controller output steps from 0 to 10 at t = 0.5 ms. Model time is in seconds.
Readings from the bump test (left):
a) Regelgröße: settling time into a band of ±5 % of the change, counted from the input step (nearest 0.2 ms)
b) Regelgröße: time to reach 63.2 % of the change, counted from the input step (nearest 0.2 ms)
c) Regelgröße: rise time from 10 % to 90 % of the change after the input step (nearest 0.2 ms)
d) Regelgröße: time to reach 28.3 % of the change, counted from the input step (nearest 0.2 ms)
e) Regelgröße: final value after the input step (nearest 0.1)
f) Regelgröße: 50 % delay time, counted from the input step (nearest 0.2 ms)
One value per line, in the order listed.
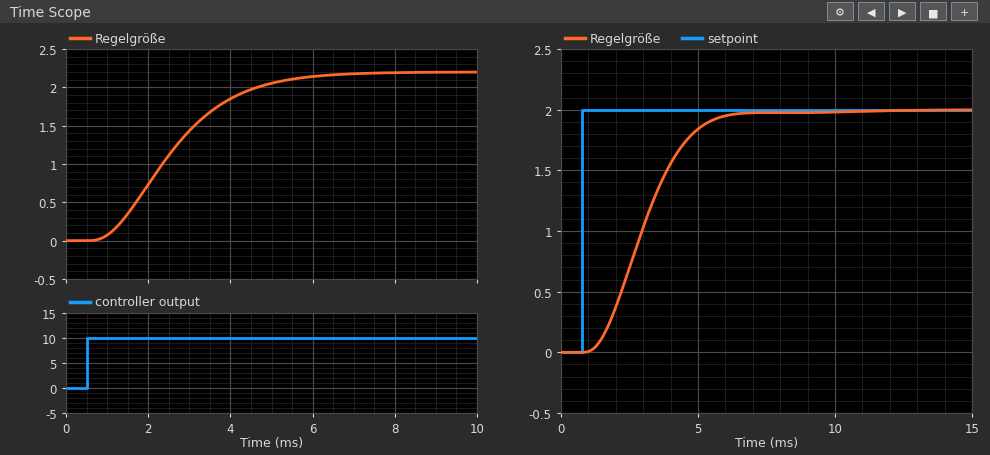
4.8 ms
2.4 ms
3.2 ms
1.4 ms
2.2
2.0 ms
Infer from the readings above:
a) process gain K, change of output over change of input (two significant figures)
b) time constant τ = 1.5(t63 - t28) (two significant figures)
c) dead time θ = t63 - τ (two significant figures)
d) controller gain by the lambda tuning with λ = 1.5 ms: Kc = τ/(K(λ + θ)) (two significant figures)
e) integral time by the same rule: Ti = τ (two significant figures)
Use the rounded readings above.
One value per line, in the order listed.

0.22
1.5 ms
0.90 ms
2.8
1.5 ms
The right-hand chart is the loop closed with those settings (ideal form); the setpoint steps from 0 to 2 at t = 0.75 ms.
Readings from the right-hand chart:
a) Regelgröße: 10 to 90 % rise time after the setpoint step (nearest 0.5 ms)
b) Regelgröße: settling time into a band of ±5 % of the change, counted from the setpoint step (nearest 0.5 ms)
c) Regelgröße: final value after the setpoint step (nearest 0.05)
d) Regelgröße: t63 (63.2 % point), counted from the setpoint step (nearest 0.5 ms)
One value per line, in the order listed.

3.0 ms
4.5 ms
2.00
2.5 ms
